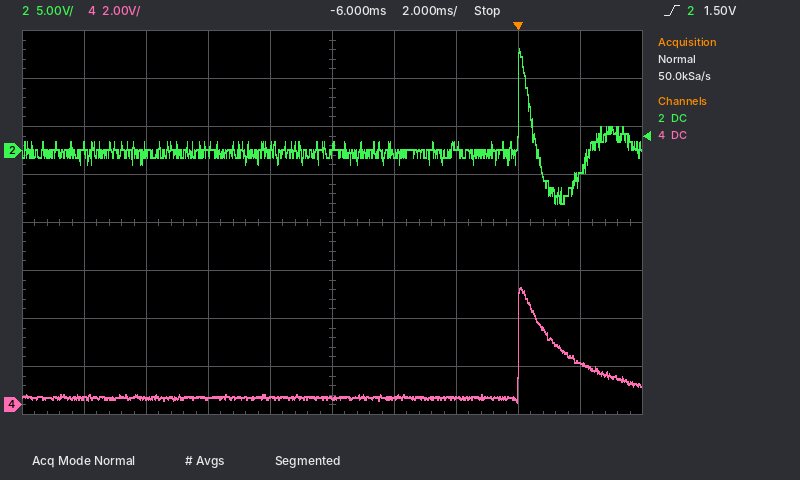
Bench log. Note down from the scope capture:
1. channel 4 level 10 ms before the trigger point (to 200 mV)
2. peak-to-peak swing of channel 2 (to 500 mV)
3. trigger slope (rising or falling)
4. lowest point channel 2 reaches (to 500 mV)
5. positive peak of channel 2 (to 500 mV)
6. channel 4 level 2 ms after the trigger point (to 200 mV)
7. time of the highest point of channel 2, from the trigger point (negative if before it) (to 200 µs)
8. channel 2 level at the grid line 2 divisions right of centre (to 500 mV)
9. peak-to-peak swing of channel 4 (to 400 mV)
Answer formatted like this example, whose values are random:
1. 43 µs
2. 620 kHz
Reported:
1. 200 mV
2. 16.0 V
3. rising
4. -5.5 V
5. 10.5 V
6. 1.8 V
7. 0.0 ms
8. 500 mV
9. 4.8 V
